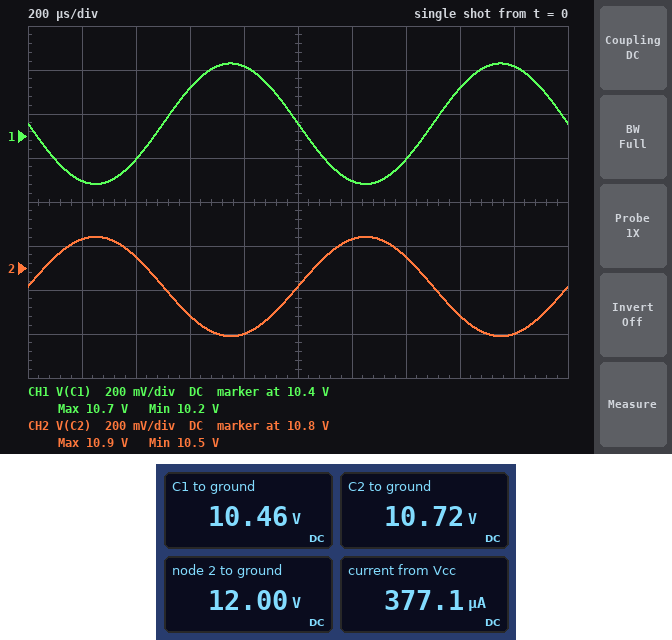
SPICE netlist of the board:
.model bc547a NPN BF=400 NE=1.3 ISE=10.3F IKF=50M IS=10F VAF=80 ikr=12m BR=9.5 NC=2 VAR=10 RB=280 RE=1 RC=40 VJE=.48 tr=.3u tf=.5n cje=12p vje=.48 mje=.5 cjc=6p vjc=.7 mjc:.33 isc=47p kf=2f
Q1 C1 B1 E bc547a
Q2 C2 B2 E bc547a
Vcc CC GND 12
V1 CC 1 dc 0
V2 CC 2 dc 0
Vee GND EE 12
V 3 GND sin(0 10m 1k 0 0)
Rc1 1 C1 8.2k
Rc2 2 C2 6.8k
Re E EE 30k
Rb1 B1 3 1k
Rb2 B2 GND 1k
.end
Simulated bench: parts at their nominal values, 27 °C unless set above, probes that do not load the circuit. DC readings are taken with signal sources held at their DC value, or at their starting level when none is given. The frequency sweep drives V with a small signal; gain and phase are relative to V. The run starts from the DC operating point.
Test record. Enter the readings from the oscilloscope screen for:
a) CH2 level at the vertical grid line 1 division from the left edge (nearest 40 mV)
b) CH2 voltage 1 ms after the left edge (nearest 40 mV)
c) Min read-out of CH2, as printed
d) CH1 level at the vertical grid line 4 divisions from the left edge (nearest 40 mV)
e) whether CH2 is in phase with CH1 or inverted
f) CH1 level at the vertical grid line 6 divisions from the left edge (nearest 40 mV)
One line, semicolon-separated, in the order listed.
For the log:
10.92 V; 10.72 V; 10.5 V; 10.72 V; inverted; 10.20 V
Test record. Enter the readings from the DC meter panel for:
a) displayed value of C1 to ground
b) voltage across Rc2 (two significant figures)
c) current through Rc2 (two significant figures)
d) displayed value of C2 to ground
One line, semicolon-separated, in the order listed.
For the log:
10.46 V; 1.3 V; 190 µA; 10.72 V
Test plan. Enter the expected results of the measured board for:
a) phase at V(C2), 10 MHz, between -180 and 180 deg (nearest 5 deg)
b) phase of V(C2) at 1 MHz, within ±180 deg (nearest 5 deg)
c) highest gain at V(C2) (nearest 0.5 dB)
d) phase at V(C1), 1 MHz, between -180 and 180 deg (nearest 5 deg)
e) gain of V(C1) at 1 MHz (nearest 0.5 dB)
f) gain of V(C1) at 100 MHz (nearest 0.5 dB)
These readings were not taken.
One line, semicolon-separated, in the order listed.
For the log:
-90 deg; -55 deg; 27.0 dB; 125 deg; 24.5 dB; -6.0 dB
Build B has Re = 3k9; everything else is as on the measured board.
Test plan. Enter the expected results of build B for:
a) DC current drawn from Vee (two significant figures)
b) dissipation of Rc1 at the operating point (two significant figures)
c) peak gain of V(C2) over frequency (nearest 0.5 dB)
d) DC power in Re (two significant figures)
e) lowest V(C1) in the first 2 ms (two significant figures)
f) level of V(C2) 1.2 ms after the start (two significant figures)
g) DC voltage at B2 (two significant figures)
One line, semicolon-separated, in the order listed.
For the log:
2.9 mA; 17 mW; 41.0 dB; 33 mW; -490 mV; 2.7 V; -8.1 mV
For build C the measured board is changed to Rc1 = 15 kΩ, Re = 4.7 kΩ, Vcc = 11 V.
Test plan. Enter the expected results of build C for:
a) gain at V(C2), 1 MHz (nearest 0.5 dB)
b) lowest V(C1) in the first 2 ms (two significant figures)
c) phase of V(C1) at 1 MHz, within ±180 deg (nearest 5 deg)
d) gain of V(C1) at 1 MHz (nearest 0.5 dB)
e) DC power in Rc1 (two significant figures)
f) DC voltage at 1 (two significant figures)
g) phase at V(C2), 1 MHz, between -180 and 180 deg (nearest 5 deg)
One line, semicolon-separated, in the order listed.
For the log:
12.5 dB; -600 mV; 55 deg; -11.0 dB; 9.0 mW; 11 V; -30 deg
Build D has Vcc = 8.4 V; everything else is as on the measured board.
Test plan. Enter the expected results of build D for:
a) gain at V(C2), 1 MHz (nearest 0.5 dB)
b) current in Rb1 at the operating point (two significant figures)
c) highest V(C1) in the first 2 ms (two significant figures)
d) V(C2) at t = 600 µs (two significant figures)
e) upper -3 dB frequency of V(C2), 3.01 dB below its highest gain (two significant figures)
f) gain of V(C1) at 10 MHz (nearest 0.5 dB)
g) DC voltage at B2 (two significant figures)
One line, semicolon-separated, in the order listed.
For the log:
22.0 dB; 1.3 µA; 7.1 V; 7.0 V; 670 kHz; 6.0 dB; -1.3 mV
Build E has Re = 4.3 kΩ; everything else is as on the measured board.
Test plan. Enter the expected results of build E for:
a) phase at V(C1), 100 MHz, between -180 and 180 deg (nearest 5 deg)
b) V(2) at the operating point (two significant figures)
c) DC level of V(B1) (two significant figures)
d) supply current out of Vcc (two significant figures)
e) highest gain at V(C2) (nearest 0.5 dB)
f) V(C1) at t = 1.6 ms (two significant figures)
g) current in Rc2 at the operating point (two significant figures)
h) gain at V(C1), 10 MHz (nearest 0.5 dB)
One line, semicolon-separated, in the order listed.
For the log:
15 deg; 12 V; -7.4 mV; 2.6 mA; 40.5 dB; 2.1 V; 1.3 mA; 5.0 dB
